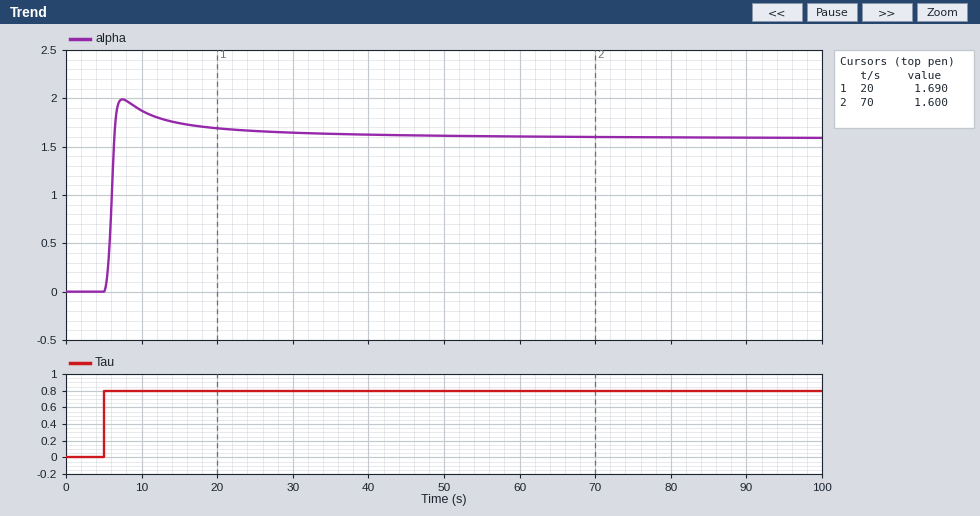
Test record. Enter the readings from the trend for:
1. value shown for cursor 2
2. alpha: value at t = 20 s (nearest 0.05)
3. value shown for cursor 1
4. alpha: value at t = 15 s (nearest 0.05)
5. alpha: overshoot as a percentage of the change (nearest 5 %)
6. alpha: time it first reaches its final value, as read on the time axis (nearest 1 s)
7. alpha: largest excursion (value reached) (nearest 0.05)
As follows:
1.600
1.70
1.690
1.75
25 %
6 s
2.00
